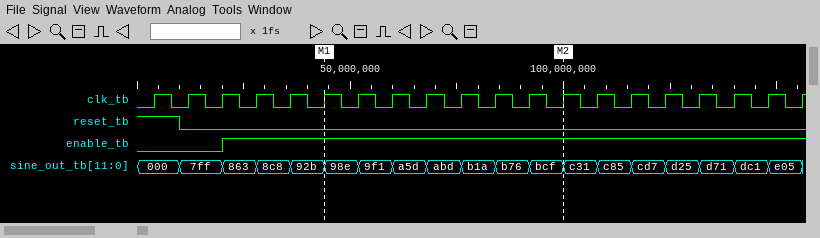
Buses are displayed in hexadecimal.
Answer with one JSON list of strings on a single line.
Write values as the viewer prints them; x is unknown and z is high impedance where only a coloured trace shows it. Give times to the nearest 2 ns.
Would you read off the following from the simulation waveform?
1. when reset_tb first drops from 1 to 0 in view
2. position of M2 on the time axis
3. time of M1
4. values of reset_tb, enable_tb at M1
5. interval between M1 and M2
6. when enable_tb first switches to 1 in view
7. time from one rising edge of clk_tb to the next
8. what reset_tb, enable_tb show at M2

["10 ns", "100 ns", "44 ns", "reset_tb=0, enable_tb=1", "56 ns", "20 ns", "8 ns", "reset_tb=0, enable_tb=1"]
